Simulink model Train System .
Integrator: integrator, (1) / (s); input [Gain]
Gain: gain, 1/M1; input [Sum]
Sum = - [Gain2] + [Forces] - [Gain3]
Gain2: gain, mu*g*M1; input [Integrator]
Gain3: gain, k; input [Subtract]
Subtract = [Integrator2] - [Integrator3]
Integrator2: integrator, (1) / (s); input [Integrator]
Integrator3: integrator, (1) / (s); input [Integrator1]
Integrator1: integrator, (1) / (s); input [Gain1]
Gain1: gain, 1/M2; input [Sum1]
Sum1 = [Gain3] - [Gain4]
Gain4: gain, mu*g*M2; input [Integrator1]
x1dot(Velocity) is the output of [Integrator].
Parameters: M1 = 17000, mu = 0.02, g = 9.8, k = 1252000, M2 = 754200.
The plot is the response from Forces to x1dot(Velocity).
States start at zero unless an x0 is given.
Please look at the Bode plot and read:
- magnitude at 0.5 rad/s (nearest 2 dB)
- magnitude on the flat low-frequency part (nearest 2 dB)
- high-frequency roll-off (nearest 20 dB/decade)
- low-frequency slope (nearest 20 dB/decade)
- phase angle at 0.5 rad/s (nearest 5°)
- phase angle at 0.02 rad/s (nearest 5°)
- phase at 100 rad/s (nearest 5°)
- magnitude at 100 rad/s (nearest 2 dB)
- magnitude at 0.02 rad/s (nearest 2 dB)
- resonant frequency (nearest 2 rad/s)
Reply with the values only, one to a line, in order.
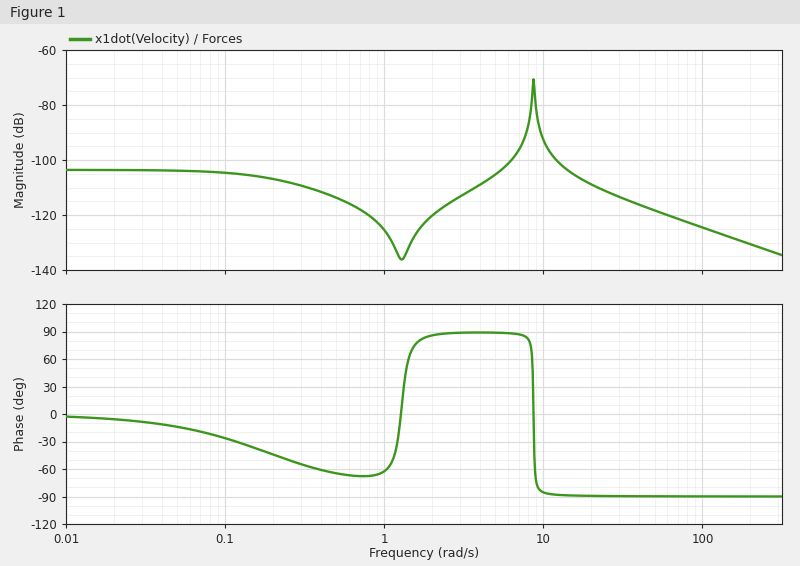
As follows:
-114 dB
-104 dB
-20 dB/decade
0 dB/decade
-65°
-5°
-90°
-124 dB
-104 dB
8 rad/s
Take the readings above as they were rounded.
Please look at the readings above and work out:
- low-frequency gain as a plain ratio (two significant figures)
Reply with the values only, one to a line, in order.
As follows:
0.0000063
